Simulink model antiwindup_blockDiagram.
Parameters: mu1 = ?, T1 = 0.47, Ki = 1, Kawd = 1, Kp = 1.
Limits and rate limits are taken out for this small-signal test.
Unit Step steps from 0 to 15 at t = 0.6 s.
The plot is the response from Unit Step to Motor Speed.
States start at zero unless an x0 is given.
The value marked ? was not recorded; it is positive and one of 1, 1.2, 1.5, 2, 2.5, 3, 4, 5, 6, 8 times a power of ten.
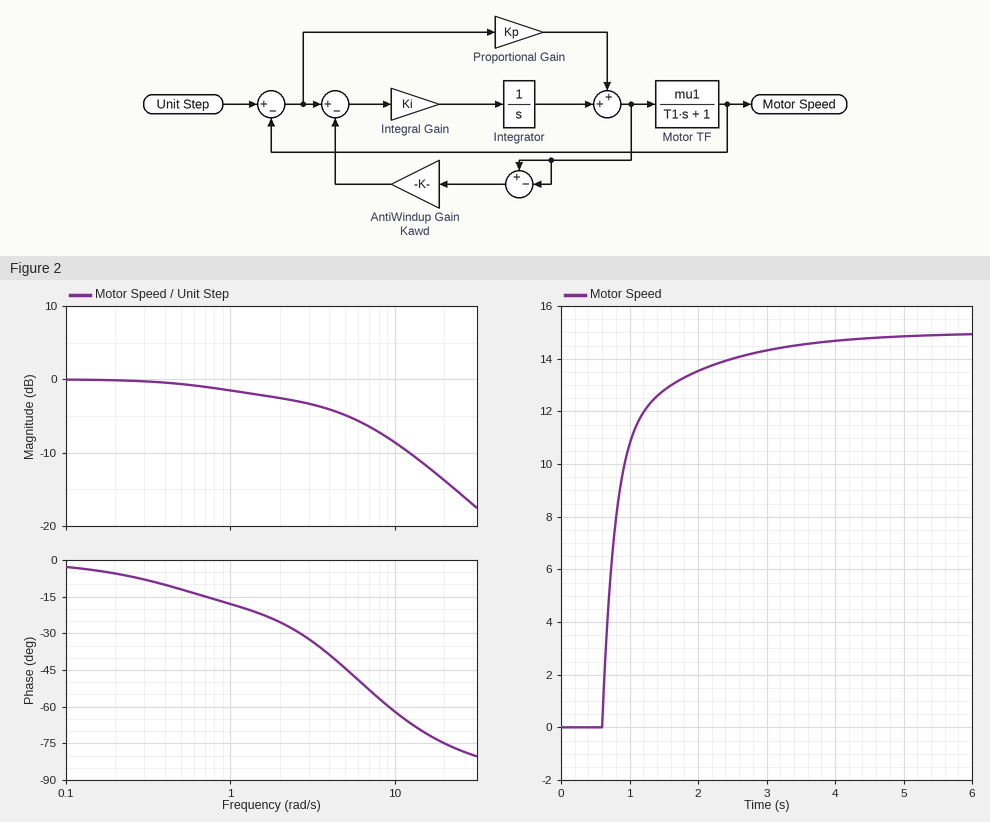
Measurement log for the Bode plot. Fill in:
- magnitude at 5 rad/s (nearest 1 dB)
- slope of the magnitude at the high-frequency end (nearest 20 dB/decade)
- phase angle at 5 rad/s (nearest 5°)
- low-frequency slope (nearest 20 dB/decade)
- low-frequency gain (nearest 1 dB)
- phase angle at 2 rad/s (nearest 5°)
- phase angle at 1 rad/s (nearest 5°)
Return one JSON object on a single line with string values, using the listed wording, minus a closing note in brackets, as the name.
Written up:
{"magnitude at 5 rad/s": "-5 dB", "slope of the magnitude at the high-frequency end": "-20 dB/decade", "phase angle at 5 rad/s": "-45°", "low-frequency slope": "0 dB/decade", "low-frequency gain": "0 dB", "phase angle at 2 rad/s": "-25°", "phase angle at 1 rad/s": "-20°"}
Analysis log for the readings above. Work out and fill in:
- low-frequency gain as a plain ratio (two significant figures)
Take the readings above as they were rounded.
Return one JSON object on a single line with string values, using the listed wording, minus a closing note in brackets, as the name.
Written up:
{"low-frequency gain as a plain ratio": "1.0"}
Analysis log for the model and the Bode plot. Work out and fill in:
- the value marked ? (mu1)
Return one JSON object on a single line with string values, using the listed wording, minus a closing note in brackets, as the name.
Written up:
{"the value marked ?": "2"}
